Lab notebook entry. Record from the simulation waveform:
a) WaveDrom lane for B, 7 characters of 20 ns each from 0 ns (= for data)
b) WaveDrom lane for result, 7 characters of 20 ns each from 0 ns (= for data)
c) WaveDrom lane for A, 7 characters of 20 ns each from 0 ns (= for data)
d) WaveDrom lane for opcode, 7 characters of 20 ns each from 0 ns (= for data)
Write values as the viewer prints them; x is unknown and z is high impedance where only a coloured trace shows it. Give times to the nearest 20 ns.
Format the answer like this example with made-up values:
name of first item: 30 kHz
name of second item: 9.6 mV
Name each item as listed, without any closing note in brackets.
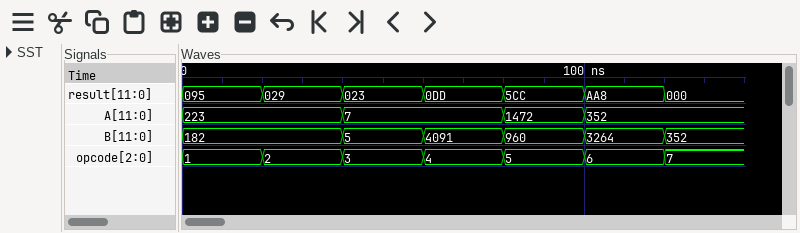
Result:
WaveDrom lane for B, 7 characters of 20 ns each from 0 ns: {name: 'B', wave: '=.=====', data: '182 5 4091 960 3264 352'}
WaveDrom lane for result, 7 characters of 20 ns each from 0 ns: {name: 'result', wave: '=======', data: '095 029 023 0DD 5CC AA8 000'}
WaveDrom lane for A, 7 characters of 20 ns each from 0 ns: {name: 'A', wave: '=.=.==.', data: '223 7 1472 352'}
WaveDrom lane for opcode, 7 characters of 20 ns each from 0 ns: {name: 'opcode', wave: '=======', data: '1 2 3 4 5 6 7'}
